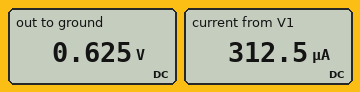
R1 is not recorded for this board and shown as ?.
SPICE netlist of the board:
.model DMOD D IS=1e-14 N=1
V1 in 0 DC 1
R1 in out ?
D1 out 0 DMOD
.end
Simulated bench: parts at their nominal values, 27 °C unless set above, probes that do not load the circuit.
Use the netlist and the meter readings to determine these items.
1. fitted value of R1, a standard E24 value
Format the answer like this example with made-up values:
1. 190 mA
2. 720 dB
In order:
1. 1.2 kΩ
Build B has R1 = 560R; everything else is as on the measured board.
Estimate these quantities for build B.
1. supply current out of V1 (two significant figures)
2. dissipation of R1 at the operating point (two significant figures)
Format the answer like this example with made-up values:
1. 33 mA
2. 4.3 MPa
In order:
1. 640 µA
2. 230 µW
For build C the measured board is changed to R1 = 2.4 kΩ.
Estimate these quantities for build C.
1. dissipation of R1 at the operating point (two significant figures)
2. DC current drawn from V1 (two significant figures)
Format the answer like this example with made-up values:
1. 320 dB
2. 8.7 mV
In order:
1. 64 µW
2. 160 µA
